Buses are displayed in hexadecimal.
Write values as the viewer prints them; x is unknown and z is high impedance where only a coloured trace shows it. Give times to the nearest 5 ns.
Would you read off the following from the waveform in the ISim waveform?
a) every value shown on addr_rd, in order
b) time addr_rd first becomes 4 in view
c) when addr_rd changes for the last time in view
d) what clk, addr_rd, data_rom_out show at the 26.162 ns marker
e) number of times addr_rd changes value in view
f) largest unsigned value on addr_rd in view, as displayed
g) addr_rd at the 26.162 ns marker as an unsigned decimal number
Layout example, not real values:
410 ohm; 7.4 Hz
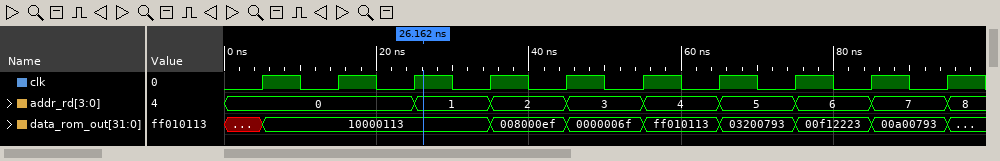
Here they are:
0, 1, 2, 3, 4, 5, 6, 7, 8; 55 ns; 95 ns; clk=1, addr_rd=1, data_rom_out=10000113; 8; 8; 1
